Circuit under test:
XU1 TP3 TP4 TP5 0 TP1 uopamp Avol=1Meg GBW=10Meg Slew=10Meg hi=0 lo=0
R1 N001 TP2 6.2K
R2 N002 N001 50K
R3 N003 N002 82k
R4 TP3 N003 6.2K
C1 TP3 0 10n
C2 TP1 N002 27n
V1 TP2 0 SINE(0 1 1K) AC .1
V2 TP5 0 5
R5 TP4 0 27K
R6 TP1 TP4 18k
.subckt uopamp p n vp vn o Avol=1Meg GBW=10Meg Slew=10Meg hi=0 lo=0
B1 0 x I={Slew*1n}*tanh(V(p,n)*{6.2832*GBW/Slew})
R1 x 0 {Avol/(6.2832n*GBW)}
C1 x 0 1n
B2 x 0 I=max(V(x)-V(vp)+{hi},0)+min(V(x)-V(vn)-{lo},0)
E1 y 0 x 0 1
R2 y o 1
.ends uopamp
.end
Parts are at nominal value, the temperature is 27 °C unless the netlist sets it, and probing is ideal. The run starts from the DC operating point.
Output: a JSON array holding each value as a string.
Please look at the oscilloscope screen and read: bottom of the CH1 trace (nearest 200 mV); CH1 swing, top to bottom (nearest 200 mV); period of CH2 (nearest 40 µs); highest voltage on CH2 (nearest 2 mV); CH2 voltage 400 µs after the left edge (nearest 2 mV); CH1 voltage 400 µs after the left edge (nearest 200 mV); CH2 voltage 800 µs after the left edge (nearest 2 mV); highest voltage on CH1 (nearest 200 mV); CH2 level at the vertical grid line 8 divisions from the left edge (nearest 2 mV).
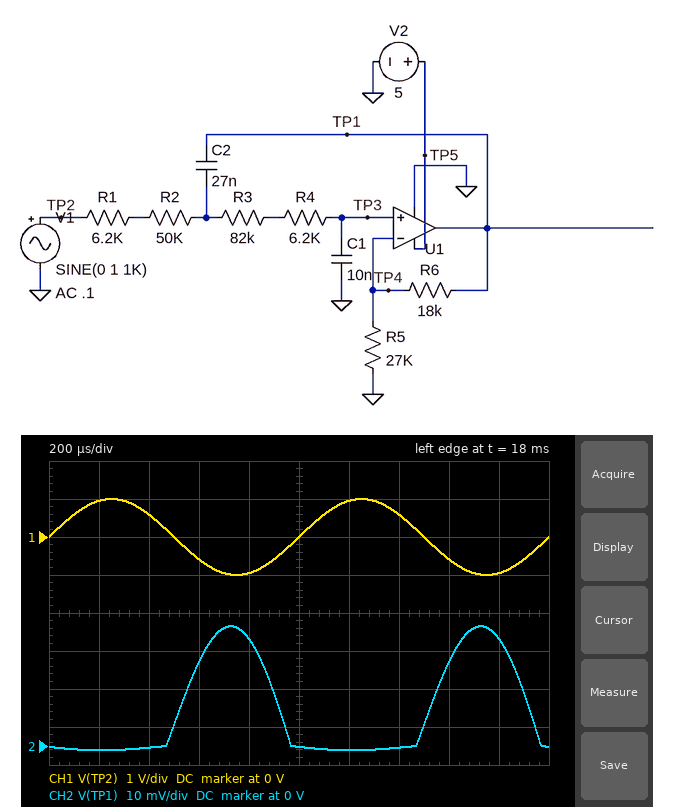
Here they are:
["-1.0 V", "2.0 V", "1.00 ms", "32 mV", "0 V", "600 mV", "28 mV", "1.0 V", "22 mV"]
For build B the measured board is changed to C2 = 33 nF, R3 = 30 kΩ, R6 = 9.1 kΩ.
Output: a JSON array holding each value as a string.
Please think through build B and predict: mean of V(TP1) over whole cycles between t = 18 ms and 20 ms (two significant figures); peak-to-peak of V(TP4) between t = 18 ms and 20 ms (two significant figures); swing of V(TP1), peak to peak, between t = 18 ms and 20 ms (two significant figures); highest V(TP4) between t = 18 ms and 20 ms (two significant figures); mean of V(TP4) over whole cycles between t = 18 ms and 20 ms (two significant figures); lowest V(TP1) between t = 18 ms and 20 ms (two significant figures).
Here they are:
["15 mV", "38 mV", "51 mV", "37 mV", "11 mV", "-2.1 mV"]
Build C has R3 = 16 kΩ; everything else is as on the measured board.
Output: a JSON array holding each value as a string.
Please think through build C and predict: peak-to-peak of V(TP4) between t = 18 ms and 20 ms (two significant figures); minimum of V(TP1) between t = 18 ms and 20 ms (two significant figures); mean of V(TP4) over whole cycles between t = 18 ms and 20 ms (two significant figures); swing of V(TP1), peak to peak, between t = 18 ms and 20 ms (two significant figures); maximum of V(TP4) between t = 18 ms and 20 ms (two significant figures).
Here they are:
["74 mV", "-3.9 mV", "21 mV", "120 mV", "72 mV"]
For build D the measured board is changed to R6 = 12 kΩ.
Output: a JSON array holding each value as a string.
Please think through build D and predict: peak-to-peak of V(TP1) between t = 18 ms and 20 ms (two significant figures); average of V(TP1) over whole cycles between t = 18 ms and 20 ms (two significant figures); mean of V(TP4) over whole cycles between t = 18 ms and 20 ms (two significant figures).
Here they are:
["28 mV", "8.3 mV", "5.7 mV"]
